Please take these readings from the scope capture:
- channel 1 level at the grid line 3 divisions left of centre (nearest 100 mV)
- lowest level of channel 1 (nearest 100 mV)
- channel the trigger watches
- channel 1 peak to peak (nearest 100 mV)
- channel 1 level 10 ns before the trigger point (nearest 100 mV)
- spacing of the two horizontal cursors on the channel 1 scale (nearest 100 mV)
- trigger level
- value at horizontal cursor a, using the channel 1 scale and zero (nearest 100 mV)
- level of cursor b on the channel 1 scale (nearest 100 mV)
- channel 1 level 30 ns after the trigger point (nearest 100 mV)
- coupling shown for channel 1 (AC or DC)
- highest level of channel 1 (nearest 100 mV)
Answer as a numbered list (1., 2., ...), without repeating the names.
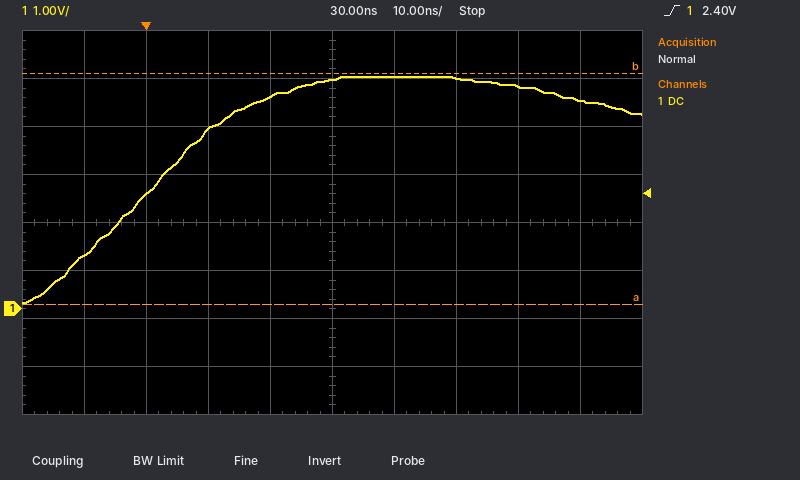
1. 2.4 V
2. 100 mV
3. channel 1
4. 4.7 V
5. 1.1 V
6. 4.8 V
7. 2.40 V
8. 100 mV
9. 4.9 V
10. 4.8 V
11. DC
12. 4.8 V
